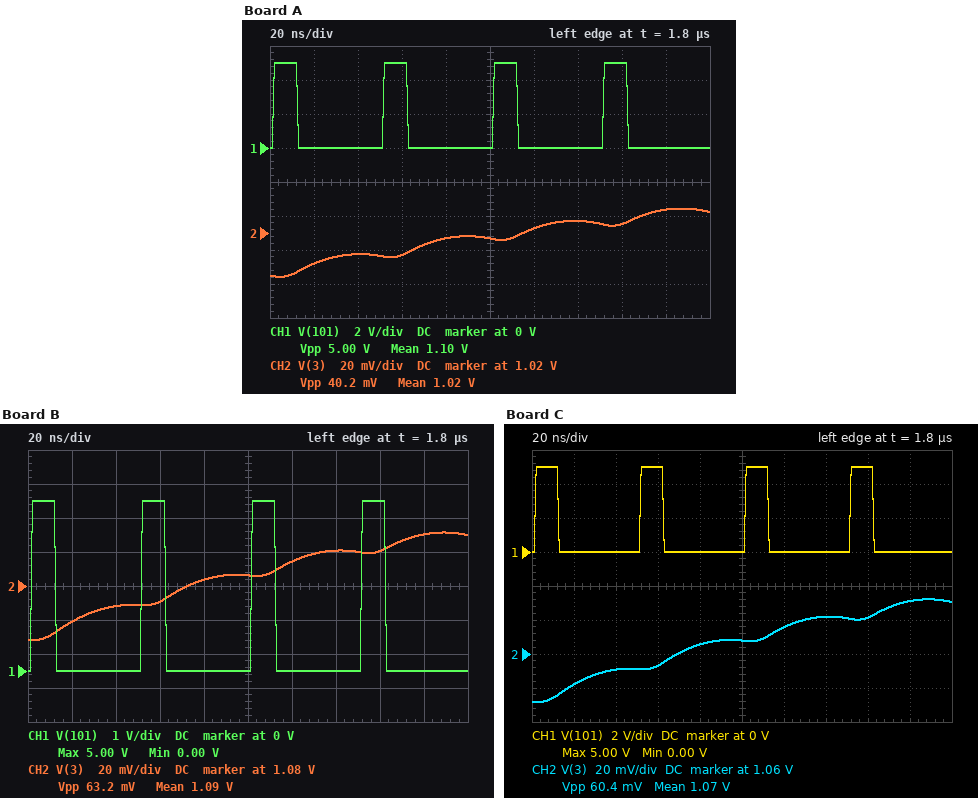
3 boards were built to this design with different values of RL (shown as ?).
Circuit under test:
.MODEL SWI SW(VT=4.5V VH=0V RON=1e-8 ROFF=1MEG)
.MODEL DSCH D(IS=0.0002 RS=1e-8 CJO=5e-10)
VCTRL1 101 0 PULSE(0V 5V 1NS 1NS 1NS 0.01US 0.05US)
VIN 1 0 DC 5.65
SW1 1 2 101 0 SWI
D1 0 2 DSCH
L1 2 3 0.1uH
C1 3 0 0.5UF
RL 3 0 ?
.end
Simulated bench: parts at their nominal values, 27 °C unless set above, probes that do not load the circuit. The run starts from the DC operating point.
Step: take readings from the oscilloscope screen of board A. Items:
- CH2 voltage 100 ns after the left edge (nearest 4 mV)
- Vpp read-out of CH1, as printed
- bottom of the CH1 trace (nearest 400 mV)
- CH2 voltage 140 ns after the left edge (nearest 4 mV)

1.016 V
5.00 V
0 V
1.028 V
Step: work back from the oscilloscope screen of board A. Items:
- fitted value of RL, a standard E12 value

0.68 Ω
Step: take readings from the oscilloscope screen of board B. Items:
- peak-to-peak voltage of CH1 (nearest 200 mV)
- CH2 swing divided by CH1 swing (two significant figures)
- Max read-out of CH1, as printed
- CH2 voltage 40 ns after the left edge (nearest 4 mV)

5.0 V
0.013
5.00 V
1.068 V
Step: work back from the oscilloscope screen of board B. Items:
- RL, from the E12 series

1.2 Ω
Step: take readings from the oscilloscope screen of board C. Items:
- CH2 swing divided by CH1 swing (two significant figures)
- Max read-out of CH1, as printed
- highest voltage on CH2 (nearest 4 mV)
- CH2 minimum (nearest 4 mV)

0.012
5.00 V
1.092 V
1.032 V
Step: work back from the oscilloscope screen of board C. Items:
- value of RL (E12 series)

1 Ω
